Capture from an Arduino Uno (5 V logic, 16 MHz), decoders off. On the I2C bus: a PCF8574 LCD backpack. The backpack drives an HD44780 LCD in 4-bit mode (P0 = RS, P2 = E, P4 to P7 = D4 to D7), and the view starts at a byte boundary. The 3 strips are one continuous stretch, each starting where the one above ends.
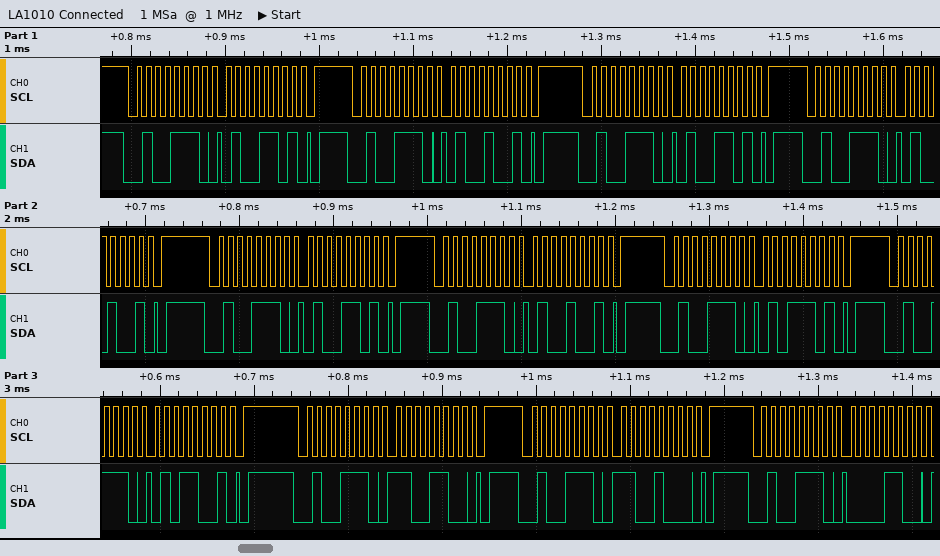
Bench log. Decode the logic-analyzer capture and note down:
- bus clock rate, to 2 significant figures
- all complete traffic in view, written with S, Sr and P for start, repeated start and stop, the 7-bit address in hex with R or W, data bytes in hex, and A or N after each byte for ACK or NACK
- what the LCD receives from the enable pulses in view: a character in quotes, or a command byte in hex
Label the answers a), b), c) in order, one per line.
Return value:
a) 100 kHz
b) S 27W A 4D A P S 27W A 49 A P S 27W A 4D A P S 27W A 49 A P S 27W A 4D A P S 27W A 49 A P S 27W A 5D A P S 27W A 59 A P S 27W A CC A P S 27W A C8 A P S 27W A 0C A
c) 'D' 'E'
